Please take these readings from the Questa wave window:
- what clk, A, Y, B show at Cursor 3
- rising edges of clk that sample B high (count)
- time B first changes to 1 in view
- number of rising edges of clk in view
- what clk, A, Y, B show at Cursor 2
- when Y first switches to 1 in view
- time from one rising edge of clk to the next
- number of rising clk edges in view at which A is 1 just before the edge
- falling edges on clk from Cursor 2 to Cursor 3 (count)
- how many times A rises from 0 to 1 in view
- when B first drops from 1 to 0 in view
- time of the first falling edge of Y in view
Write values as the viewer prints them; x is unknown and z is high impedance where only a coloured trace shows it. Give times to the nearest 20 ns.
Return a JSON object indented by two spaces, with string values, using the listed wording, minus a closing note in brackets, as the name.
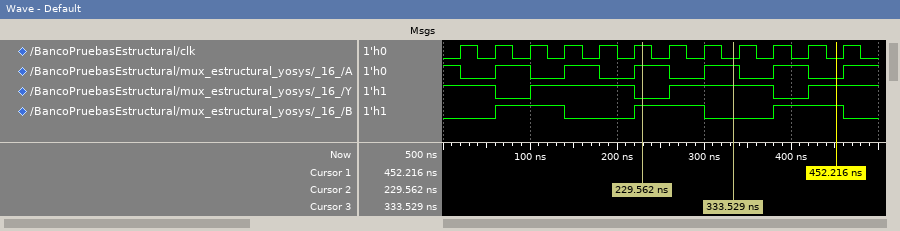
{
  "what clk, A, Y, B show at Cursor 3": "clk=0, A=1, Y=1, B=0",
  "rising edges of clk that sample B high": "6",
  "time B first changes to 1 in view": "60 ns",
  "number of rising edges of clk in view": "12",
  "what clk, A, Y, B show at Cursor 2": "clk=1, A=1, Y=0, B=1",
  "when Y first switches to 1 in view": "100 ns",
  "time from one rising edge of clk to the next": "40 ns",
  "number of rising clk edges in view at which A is 1 just before the edge": "6",
  "falling edges on clk from Cursor 2 to Cursor 3": "3",
  "how many times A rises from 0 to 1 in view": "6",
  "when B first drops from 1 to 0 in view": "140 ns",
  "time of the first falling edge of Y in view": "60 ns"
}
